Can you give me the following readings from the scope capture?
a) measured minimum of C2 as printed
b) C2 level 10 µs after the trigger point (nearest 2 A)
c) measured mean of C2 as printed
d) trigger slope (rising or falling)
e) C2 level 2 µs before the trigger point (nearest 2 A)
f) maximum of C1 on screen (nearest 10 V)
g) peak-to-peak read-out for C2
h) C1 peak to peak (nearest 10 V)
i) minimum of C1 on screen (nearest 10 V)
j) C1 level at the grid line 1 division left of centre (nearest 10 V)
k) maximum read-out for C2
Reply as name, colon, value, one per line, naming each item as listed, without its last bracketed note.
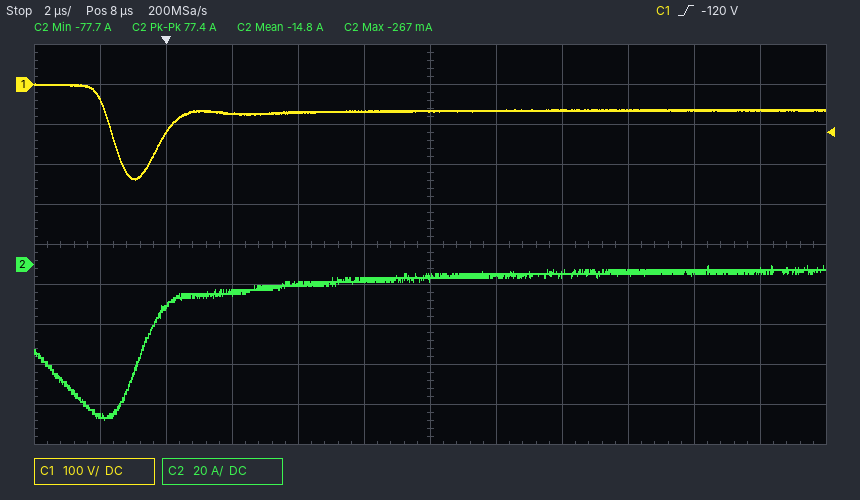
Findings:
measured minimum of C2 as printed: -77.7 A
C2 level 10 µs after the trigger point: -6 A
measured mean of C2 as printed: -14.8 A
trigger slope: rising
C2 level 2 µs before the trigger point: -76 A
maximum of C1 on screen: 0 V
peak-to-peak read-out for C2: 77.4 A
C1 peak to peak: 240 V
minimum of C1 on screen: -240 V
C1 level at the grid line 1 division left of centre: -70 V
maximum read-out for C2: -267 mA
